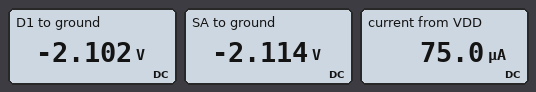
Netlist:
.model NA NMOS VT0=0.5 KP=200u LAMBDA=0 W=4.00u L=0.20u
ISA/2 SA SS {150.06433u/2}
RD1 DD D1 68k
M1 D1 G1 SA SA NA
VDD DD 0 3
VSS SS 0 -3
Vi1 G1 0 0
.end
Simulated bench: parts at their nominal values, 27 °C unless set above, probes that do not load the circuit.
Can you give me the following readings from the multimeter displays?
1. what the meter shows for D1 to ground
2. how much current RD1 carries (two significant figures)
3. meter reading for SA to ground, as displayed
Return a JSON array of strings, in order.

["-2.102 V", "75 µA", "-2.114 V"]
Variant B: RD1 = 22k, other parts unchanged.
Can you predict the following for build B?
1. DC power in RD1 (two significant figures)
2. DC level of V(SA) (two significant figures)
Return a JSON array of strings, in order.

["120 µW", "-690 mV"]
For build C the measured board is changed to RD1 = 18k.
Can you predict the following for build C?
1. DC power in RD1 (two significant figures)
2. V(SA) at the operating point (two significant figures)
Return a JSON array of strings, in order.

["100 µW", "-690 mV"]
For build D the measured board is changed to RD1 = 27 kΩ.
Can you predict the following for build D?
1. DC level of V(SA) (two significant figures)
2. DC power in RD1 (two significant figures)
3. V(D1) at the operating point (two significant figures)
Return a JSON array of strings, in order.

["-690 mV", "150 µW", "970 mV"]
